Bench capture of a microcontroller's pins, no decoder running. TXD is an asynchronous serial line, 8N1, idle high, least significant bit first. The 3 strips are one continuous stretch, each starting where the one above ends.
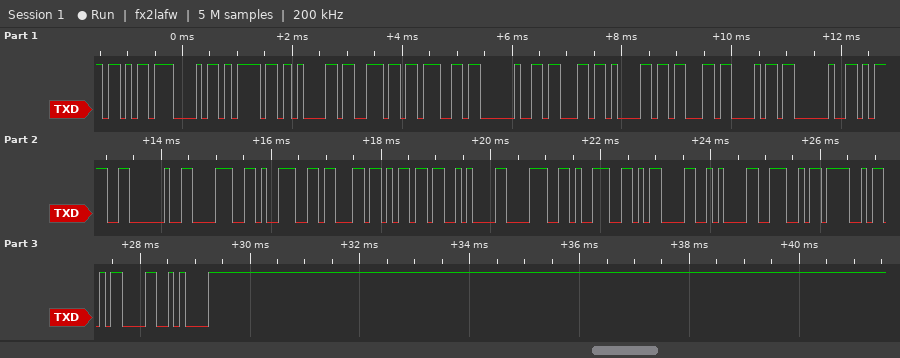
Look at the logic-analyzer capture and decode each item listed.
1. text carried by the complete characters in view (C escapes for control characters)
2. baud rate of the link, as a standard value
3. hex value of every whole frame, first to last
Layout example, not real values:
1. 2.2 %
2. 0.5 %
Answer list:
1. "khoang cach = 89cm\n89\r\nNO\r\n"
2. 9600 baud
3. 6B 68 6F 61 6E 67 20 63 61 63 68 20 3D 20 38 39 63 6D 0A 38 39 0D 0A 4E 4F 0D 0A
